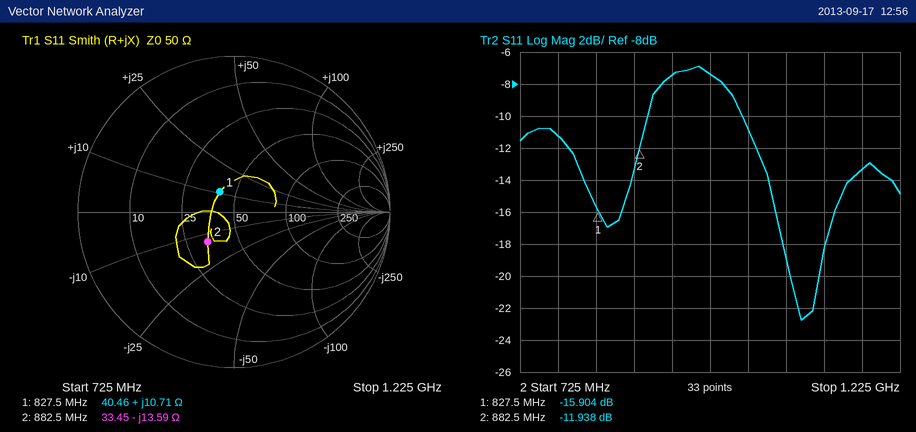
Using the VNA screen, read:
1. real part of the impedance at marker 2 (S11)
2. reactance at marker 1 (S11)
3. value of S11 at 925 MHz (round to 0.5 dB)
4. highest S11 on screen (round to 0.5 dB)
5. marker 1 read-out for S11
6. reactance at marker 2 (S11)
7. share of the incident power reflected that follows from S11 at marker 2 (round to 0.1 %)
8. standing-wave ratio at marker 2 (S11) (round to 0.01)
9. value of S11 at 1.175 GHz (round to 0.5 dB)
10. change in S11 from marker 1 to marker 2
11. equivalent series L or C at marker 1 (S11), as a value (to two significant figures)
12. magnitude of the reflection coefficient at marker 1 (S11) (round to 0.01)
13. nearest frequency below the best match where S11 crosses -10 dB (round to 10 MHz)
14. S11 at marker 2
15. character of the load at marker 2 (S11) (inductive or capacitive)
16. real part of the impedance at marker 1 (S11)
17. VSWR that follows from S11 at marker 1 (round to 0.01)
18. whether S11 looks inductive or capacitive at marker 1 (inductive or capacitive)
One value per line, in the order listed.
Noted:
33.45 Ω
+10.71 Ω
-7.5 dB
-7.0 dB
-15.904 dB
-13.59 Ω
6.4 %
1.68
-13.5 dB
3.966 dB
2.1 nH
0.16
1.02 GHz
-11.938 dB
capacitive
40.46 Ω
1.38
inductive
